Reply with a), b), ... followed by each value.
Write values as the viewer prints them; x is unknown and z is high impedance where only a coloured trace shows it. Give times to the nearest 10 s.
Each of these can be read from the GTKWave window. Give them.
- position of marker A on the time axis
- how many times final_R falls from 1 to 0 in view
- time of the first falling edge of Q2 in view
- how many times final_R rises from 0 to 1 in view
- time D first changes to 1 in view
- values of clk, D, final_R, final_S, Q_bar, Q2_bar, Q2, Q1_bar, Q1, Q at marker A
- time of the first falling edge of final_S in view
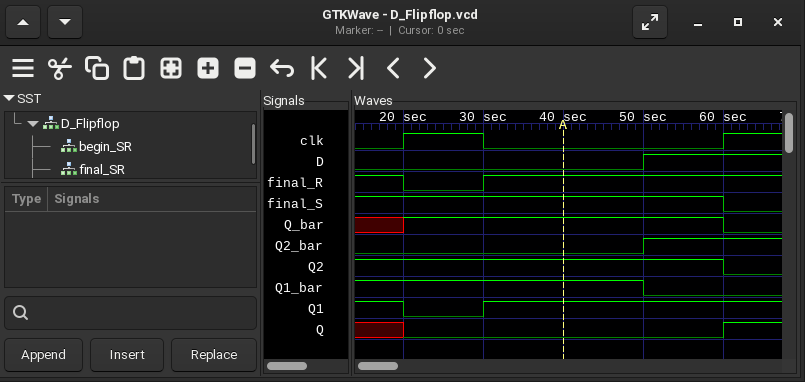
a) 40 s
b) 1
c) 60 s
d) 1
e) 50 s
f) clk=0, D=0, final_R=1, final_S=1, Q_bar=1, Q2_bar=0, Q2=1, Q1_bar=1, Q1=1, Q=0
g) 60 s
